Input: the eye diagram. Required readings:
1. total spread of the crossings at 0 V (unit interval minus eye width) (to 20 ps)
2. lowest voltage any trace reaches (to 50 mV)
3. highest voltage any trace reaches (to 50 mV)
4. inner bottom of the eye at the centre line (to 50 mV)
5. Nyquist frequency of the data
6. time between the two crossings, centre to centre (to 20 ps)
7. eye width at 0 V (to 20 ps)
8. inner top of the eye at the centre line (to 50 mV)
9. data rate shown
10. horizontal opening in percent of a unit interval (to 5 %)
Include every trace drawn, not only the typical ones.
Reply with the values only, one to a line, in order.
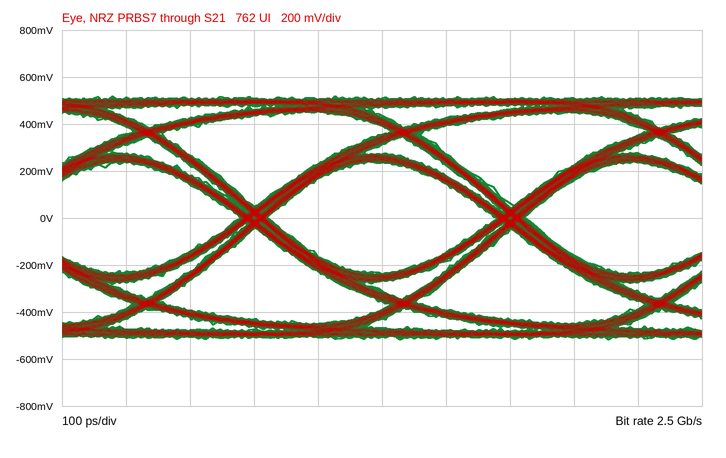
40 ps
-500 mV
500 mV
-250 mV
1.25 GHz
400 ps
360 ps
250 mV
2.5 Gb/s
90 %
